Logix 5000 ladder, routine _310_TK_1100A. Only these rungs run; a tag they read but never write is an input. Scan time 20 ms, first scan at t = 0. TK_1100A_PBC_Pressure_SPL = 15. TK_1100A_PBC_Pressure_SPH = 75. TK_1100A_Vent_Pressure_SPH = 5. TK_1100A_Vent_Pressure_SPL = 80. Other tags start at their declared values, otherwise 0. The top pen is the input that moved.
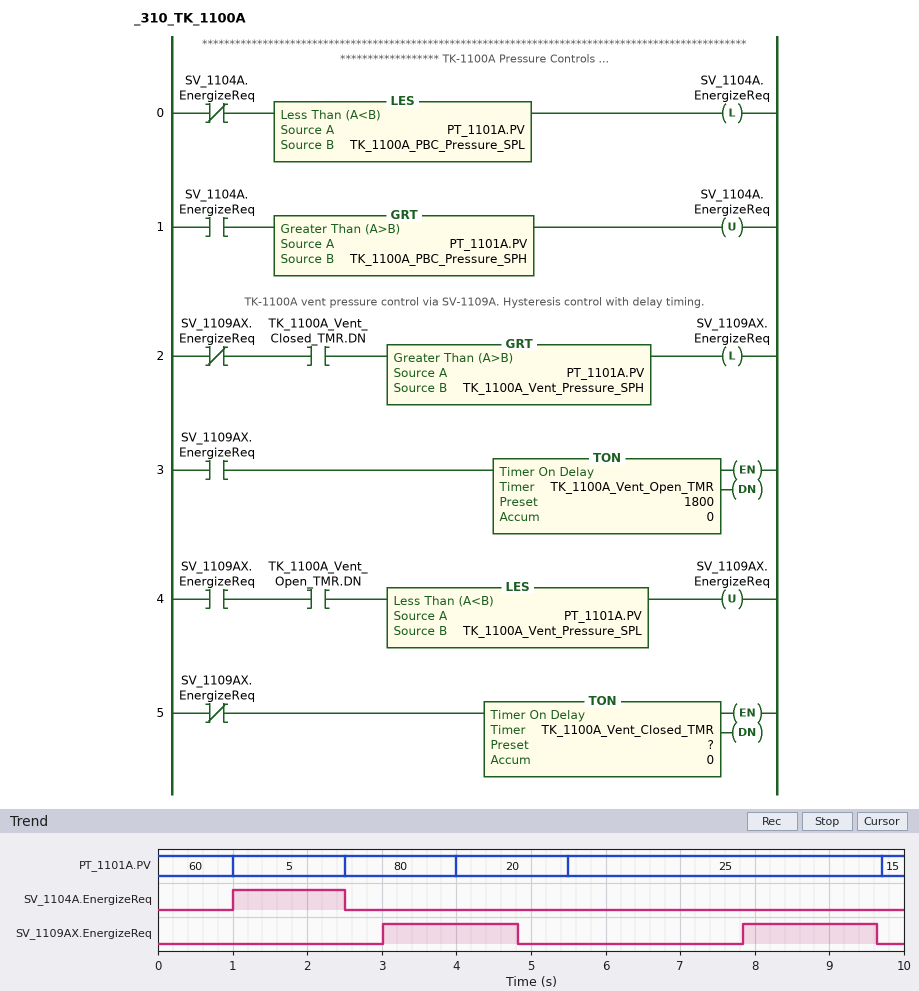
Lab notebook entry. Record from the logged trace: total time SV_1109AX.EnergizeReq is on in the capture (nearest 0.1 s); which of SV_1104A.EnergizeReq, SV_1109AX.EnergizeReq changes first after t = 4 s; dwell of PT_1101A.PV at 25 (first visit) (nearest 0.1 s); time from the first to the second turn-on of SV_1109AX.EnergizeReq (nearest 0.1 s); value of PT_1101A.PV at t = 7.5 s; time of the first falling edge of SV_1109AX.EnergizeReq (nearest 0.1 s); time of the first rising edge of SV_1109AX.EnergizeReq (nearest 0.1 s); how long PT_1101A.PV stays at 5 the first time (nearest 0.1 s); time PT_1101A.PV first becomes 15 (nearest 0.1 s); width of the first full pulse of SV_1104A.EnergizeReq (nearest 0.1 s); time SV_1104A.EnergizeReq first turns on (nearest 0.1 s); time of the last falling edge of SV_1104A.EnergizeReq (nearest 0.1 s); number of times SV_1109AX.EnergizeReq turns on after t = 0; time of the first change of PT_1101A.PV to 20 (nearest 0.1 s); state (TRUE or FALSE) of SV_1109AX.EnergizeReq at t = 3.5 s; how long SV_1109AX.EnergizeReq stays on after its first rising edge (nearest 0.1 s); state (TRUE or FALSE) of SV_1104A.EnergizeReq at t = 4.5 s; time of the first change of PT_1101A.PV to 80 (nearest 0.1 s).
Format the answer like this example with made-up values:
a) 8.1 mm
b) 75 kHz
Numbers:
a) 3.6 s
b) SV_1109AX.EnergizeReq
c) 4.2 s
d) 4.8 s
e) 25
f) 4.8 s
g) 3.0 s
h) 1.5 s
i) 9.7 s
j) 1.5 s
k) 1.0 s
l) 2.5 s
m) 2
n) 4.0 s
o) TRUE
p) 1.8 s
q) FALSE
r) 2.5 s
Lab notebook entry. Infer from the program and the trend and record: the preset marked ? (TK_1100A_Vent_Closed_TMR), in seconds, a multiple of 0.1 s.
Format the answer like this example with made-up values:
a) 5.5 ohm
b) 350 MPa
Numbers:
a) 3.0 s
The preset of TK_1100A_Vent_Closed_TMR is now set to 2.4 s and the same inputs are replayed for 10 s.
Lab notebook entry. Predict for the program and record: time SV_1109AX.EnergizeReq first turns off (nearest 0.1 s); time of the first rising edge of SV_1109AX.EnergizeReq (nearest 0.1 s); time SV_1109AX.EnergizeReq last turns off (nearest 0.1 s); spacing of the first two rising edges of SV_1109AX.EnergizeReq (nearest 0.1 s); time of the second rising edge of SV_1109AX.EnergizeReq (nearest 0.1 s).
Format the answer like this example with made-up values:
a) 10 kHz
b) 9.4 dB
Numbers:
a) 4.3 s
b) 2.5 s
c) 8.5 s
d) 4.2 s
e) 6.7 s
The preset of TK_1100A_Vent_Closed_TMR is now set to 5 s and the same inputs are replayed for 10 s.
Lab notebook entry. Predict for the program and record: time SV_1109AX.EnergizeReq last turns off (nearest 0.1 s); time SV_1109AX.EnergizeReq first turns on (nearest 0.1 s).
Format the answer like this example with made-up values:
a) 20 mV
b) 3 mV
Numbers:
a) 6.8 s
b) 5.0 s
